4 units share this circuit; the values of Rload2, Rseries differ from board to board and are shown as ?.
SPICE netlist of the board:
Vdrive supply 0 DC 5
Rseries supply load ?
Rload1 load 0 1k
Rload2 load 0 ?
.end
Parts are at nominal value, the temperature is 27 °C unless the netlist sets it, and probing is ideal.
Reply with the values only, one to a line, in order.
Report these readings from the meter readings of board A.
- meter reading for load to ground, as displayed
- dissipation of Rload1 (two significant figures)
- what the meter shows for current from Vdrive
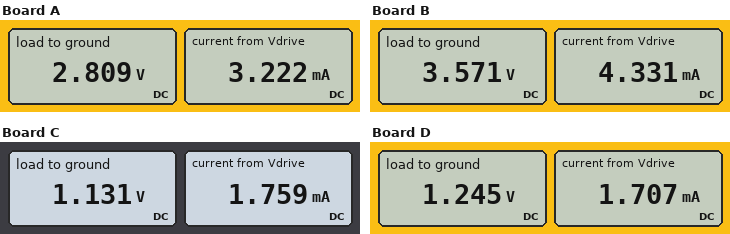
2.809 V
7.9 mW
3.222 mA
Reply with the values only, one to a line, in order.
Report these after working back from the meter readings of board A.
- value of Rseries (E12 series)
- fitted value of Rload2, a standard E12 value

680 Ω
6.8 kΩ
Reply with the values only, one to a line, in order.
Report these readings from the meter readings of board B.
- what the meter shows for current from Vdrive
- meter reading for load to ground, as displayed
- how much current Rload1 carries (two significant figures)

4.331 mA
3.571 V
3.6 mA
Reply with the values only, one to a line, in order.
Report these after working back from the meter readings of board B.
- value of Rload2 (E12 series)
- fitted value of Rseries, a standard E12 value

4.7 kΩ
330 Ω
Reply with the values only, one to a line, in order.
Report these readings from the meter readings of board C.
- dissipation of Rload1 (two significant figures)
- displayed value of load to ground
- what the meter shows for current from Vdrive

1.3 mW
1.131 V
1.759 mA
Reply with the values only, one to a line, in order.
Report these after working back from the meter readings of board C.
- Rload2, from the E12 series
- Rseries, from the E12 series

1.8 kΩ
2.2 kΩ
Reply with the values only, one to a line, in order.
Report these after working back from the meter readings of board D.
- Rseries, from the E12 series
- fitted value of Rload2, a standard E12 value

2.2 kΩ
2.7 kΩ
